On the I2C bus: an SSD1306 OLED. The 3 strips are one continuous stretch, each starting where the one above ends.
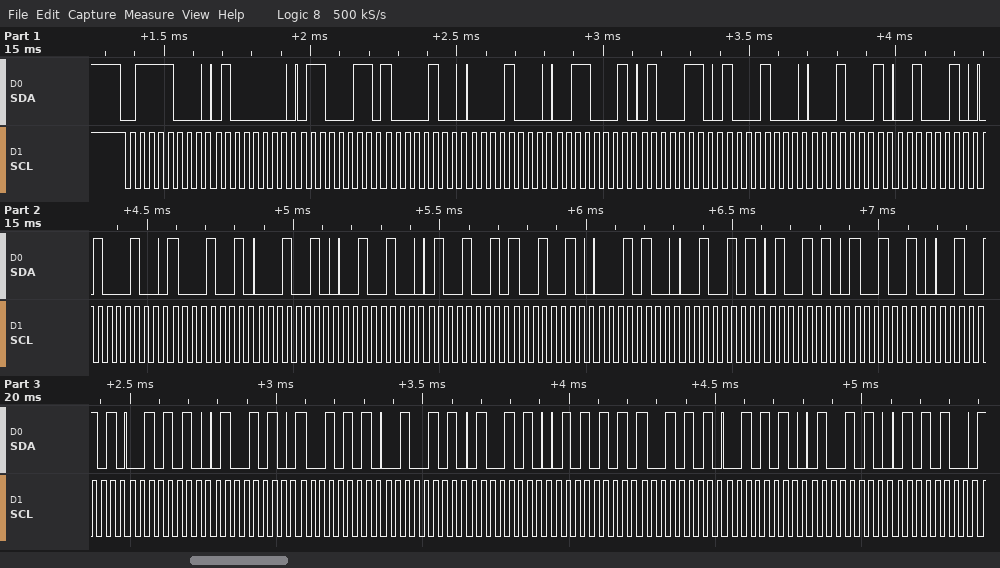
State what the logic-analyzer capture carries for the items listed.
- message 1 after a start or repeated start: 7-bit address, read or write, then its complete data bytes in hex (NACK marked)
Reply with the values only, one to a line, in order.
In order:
0x3C write: 40 63 84 08 31 46 88 11 22 44 89 12 24 49 92 14 25 4A 92 25 2A 4A 95 25 4A 55 95 2A 4A 54
